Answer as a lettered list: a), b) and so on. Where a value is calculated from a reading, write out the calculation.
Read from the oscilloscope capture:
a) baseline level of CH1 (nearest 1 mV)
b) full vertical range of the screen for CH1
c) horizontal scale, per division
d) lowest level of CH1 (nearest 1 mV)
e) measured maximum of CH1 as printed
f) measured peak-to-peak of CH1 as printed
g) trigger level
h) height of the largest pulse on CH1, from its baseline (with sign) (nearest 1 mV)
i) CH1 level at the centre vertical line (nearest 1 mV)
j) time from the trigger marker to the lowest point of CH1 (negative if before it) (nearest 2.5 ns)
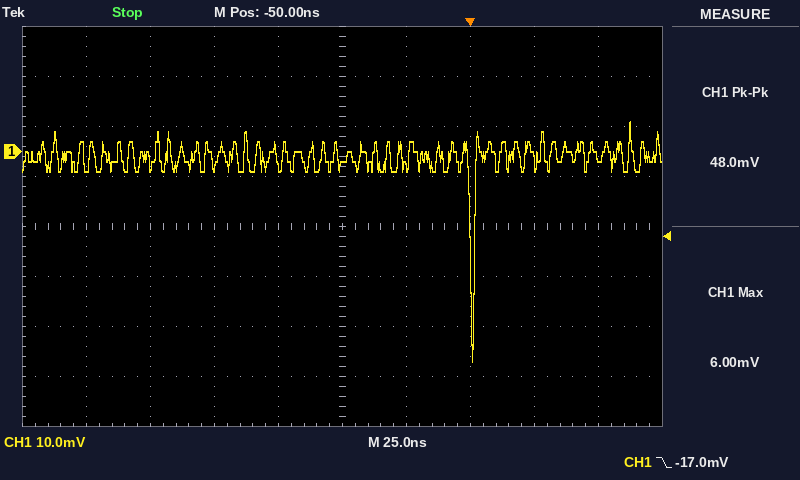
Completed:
a) -1 mV
b) 80 mV
c) 25 ns
d) -42 mV
e) 6.00 mV
f) 48.0 mV
g) -17.0 mV
h) -42 mV − (-1 mV) = -41 mV
i) -3 mV
j) 0.0 ns
